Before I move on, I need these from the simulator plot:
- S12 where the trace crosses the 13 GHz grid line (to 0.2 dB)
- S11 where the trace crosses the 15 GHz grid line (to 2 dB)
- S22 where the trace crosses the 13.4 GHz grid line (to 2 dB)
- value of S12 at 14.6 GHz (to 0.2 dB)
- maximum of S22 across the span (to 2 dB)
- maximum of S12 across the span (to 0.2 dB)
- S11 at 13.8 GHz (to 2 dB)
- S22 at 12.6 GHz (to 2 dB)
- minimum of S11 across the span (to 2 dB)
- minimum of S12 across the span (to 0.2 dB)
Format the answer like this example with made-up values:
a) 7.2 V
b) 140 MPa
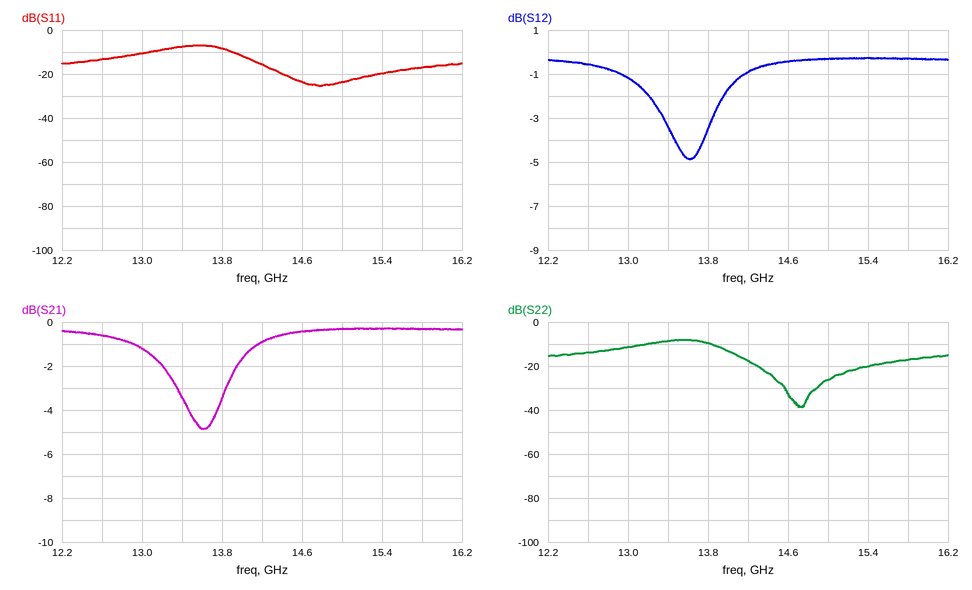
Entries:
a) -1.2 dB
b) -24 dB
c) -8 dB
d) -0.4 dB
e) -8 dB
f) -0.2 dB
g) -8 dB
h) -14 dB
i) -26 dB
j) -4.8 dB
